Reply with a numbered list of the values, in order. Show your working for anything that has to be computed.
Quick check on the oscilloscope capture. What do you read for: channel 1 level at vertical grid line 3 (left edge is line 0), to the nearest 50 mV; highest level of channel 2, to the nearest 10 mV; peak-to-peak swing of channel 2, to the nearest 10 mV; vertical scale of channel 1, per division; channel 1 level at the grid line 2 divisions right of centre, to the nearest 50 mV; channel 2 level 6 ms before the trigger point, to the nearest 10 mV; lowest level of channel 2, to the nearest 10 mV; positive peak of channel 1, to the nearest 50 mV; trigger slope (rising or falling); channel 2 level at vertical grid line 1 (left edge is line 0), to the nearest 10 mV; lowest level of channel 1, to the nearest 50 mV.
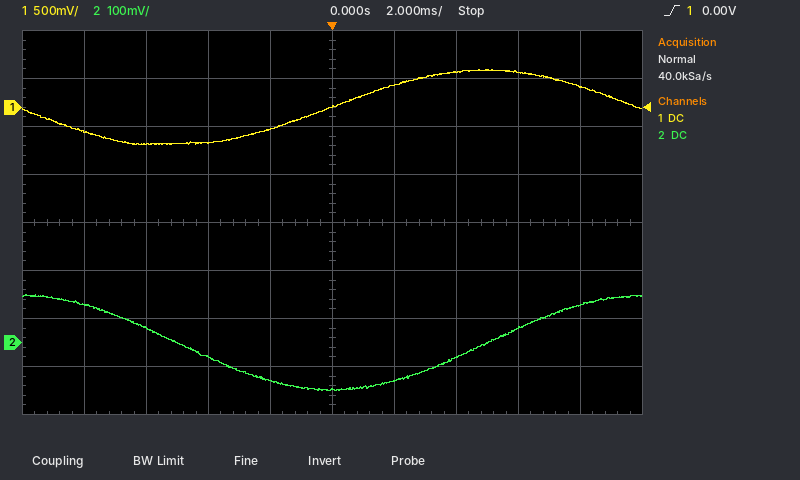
1. -350 mV
2. 100 mV
3. 100 mV − (-100 mV) = 200 mV
4. 500 mV
5. 350 mV
6. 30 mV
7. -100 mV
8. 400 mV
9. rising
10. 80 mV
11. -400 mV
